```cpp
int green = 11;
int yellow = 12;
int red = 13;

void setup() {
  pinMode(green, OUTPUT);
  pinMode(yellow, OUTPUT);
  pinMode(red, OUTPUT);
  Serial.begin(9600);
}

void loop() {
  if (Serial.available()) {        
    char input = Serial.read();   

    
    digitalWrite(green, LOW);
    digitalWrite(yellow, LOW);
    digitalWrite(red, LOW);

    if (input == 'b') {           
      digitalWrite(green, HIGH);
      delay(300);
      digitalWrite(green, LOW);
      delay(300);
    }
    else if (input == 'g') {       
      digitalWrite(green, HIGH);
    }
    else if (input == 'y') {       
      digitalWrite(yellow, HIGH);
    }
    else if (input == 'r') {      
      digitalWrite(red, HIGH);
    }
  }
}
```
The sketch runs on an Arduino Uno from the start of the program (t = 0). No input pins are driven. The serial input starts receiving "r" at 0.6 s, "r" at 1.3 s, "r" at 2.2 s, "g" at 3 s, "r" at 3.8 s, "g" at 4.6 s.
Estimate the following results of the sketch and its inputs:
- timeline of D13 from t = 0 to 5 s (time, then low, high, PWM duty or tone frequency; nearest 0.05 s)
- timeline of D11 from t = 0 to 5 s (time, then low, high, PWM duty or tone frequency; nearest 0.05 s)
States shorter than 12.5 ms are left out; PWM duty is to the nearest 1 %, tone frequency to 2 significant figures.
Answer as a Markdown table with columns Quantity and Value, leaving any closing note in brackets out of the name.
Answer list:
| Quantity | Value |
|---|---|
| timeline of D13 from t = 0 to 5 s | 0 s low; 0.6 s high; 3 s low; 3.8 s high; 4.6 s low |
| timeline of D11 from t = 0 to 5 s | 0 s low; 3 s high; 3.8 s low; 4.6 s high |
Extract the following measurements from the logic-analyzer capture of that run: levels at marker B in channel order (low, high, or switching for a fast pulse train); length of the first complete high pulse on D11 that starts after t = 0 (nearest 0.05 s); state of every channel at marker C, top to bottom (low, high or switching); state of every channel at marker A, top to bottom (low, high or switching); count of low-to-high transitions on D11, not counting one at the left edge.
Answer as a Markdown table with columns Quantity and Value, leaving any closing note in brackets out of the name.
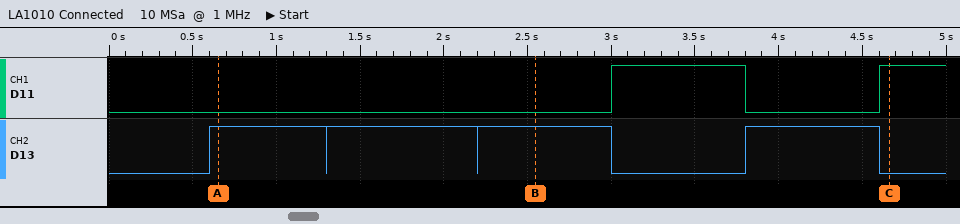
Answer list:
| Quantity | Value |
|---|---|
| levels at marker B in channel order | D11 low, D13 high |
| length of the first complete high pulse on D11 that starts after t = 0 | 0.80 s |
| state of every channel at marker C, top to bottom | D11 high, D13 low |
| state of every channel at marker A, top to bottom | D11 low, D13 high |
| count of low-to-high transitions on D11, not counting one at the left edge | 2 |
